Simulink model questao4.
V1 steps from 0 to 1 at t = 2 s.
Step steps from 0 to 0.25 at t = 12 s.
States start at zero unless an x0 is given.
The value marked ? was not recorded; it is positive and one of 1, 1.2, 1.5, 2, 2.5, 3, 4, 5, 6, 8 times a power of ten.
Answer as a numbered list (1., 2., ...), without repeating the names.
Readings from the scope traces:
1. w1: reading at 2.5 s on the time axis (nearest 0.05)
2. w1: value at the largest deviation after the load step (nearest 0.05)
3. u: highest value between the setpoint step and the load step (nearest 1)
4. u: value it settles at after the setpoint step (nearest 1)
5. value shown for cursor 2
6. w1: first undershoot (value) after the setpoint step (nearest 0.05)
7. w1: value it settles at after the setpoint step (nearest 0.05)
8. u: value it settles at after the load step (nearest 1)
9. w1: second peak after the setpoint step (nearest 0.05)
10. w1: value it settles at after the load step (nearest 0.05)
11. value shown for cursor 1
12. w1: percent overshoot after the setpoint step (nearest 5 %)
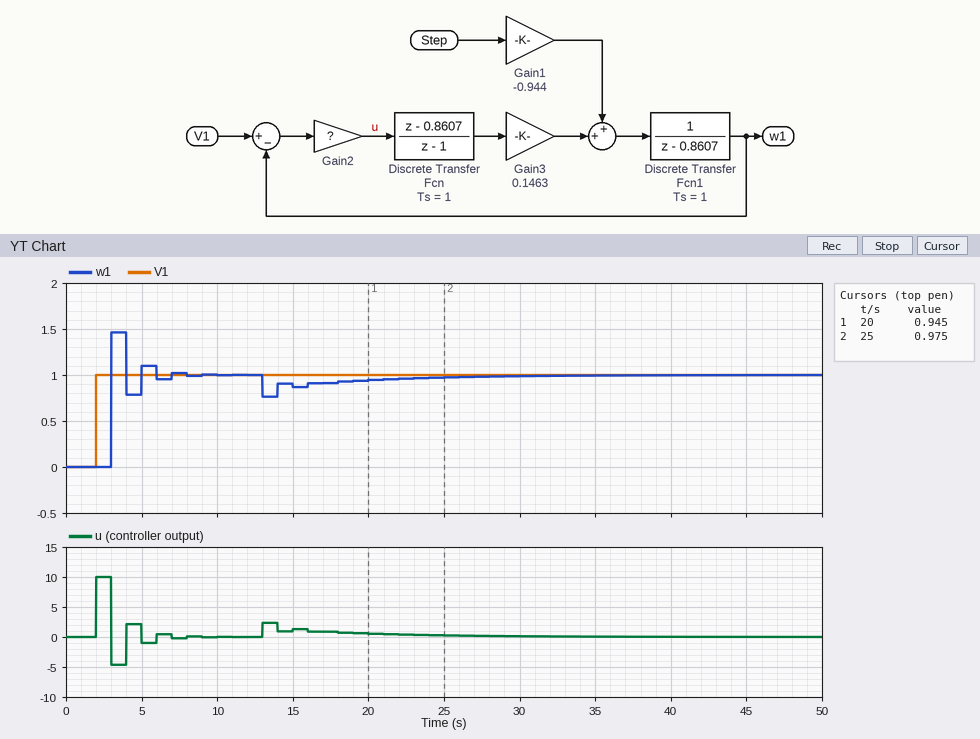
1. 0.00
2. 0.75
3. 10
4. 0
5. 0.975
6. 0.80
7. 1.00
8. 0
9. 1.10
10. 1.00
11. 0.945
12. 45 %
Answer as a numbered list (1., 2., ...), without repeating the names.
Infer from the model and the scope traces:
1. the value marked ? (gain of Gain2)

1. 10
